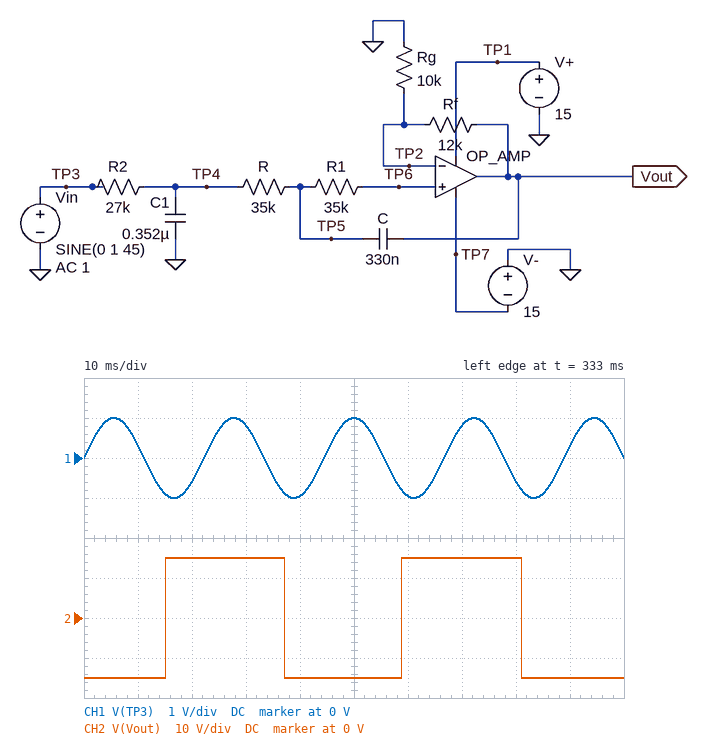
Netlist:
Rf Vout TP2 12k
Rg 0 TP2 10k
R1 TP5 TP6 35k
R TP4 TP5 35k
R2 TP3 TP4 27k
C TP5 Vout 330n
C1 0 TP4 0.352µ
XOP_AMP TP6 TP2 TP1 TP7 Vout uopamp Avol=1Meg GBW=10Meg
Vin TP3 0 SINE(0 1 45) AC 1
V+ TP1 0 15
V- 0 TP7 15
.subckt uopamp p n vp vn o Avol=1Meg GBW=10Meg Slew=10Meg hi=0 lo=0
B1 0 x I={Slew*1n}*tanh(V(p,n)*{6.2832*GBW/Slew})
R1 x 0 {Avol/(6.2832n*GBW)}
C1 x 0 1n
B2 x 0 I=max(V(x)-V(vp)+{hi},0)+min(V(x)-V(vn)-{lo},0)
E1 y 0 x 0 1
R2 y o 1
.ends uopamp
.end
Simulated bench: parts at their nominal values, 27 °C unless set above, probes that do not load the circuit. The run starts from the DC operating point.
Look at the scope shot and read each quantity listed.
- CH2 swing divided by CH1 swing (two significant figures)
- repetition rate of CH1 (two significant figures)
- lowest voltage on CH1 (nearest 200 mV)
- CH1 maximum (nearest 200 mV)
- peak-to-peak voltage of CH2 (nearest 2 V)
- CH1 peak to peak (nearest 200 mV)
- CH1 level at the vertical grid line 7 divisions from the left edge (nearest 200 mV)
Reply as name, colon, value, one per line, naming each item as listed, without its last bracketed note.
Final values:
CH2 swing divided by CH1 swing: 15
repetition rate of CH1: 45 Hz
lowest voltage on CH1: -1.0 V
CH1 maximum: 1.0 V
peak-to-peak voltage of CH2: 30 V
CH1 peak to peak: 2.0 V
CH1 level at the vertical grid line 7 divisions from the left edge: 800 mV
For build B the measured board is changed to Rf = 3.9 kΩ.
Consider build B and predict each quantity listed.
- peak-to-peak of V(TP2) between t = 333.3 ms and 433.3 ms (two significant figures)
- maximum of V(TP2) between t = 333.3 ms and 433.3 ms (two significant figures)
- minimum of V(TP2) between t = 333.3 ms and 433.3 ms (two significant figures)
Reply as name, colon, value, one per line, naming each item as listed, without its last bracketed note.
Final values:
peak-to-peak of V(TP2) between t = 333.3 ms and 433.3 ms: 22 V
maximum of V(TP2) between t = 333.3 ms and 433.3 ms: 11 V
minimum of V(TP2) between t = 333.3 ms and 433.3 ms: -11 V
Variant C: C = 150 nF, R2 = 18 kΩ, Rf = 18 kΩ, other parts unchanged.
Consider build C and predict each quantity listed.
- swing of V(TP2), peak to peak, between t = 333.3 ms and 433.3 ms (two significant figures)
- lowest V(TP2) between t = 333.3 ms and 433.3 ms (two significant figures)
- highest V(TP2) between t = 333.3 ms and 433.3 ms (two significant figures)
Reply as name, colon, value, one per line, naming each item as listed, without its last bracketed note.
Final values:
swing of V(TP2), peak to peak, between t = 333.3 ms and 433.3 ms: 11 V
lowest V(TP2) between t = 333.3 ms and 433.3 ms: -5.4 V
highest V(TP2) between t = 333.3 ms and 433.3 ms: 5.4 V
